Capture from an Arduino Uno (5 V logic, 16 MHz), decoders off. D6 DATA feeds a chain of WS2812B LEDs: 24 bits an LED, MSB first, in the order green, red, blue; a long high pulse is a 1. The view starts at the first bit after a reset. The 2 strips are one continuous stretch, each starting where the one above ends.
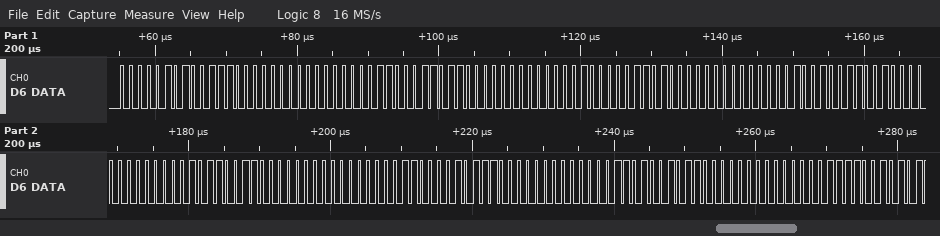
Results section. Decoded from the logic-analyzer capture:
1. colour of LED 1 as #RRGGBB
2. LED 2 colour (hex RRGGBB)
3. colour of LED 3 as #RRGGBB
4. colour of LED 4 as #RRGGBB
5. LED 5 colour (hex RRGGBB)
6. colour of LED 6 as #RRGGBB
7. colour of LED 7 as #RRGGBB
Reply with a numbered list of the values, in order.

1. #380500
2. #360600
3. #340800
4. #320900
5. #300B00
6. #2E0C00
7. #2C0D00
